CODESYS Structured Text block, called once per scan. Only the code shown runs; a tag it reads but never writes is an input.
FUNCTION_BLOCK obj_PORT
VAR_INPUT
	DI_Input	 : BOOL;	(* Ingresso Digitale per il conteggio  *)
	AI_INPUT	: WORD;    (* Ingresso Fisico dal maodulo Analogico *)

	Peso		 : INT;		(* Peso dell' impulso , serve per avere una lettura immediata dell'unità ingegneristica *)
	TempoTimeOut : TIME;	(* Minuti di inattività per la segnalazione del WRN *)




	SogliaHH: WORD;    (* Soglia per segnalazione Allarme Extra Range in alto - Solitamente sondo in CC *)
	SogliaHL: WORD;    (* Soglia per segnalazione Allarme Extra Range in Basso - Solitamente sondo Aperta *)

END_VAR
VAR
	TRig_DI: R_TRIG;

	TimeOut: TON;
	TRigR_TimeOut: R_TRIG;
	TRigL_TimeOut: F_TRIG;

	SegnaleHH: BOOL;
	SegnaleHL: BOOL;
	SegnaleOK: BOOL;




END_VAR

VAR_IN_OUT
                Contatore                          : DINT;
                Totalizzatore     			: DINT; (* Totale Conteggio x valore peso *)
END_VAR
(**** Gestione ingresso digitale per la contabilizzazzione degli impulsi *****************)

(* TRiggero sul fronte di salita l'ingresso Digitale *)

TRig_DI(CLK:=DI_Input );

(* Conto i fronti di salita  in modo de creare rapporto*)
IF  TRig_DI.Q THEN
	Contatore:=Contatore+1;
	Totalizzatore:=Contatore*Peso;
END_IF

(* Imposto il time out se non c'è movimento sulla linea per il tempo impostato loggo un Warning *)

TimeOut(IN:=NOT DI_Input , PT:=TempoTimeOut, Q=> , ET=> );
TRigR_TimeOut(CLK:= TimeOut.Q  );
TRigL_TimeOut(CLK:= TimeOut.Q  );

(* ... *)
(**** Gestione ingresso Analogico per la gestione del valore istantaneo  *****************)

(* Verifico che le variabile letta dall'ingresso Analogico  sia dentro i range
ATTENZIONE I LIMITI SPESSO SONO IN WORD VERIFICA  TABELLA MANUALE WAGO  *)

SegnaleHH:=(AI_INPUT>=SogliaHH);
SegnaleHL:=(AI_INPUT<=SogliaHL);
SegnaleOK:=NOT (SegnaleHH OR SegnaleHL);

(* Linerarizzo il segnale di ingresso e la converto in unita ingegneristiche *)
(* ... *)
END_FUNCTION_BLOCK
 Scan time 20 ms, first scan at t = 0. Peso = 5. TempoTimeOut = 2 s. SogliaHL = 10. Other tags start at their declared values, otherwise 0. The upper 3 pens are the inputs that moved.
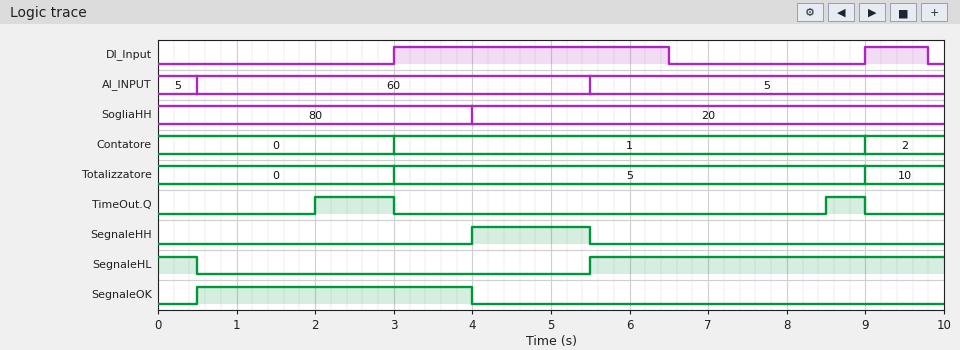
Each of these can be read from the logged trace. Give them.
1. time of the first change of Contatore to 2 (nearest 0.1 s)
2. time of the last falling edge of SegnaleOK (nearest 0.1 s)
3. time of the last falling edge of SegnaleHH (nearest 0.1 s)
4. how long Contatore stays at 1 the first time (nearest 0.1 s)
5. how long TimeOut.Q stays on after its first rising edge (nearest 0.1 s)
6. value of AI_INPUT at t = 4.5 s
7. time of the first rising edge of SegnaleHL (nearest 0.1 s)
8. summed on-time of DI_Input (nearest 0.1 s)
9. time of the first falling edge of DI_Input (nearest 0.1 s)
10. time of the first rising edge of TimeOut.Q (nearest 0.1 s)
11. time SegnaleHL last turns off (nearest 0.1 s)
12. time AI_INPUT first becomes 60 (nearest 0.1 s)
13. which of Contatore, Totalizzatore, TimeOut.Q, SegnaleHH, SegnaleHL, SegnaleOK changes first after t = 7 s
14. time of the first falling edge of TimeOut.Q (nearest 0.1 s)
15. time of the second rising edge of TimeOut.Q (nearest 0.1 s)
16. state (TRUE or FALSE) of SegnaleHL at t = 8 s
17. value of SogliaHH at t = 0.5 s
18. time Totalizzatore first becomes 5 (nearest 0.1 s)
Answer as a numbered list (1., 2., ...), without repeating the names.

1. 9.0 s
2. 4.0 s
3. 5.5 s
4. 6.0 s
5. 1.0 s
6. 60
7. 5.5 s
8. 4.3 s
9. 6.5 s
10. 2.0 s
11. 0.5 s
12. 0.5 s
13. TimeOut.Q
14. 3.0 s
15. 8.5 s
16. TRUE
17. 80
18. 3.0 s
